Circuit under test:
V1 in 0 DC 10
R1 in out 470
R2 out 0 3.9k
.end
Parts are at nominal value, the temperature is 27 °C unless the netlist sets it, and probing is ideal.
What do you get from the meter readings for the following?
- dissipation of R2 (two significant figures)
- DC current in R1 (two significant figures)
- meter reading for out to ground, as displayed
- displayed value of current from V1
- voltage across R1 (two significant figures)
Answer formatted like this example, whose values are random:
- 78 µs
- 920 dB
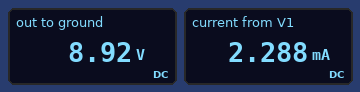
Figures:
- 20 mW
- 2.3 mA
- 8.92 V
- 2.288 mA
- 1.1 V
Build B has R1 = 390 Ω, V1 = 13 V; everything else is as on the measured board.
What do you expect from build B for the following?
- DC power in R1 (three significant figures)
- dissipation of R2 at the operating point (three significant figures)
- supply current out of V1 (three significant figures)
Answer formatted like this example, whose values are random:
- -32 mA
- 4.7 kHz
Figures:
- 3.58 mW
- 35.8 mW
- 3.03 mA
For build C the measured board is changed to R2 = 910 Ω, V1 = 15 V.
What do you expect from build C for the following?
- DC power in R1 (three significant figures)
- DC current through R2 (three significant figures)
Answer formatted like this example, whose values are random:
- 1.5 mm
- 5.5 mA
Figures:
- 55.5 mW
- 10.9 mA
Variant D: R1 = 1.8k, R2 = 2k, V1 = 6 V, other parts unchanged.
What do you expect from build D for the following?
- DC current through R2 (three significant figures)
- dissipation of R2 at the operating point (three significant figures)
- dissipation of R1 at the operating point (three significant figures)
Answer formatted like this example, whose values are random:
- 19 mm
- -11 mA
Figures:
- 1.58 mA
- 4.99 mW
- 4.49 mW
